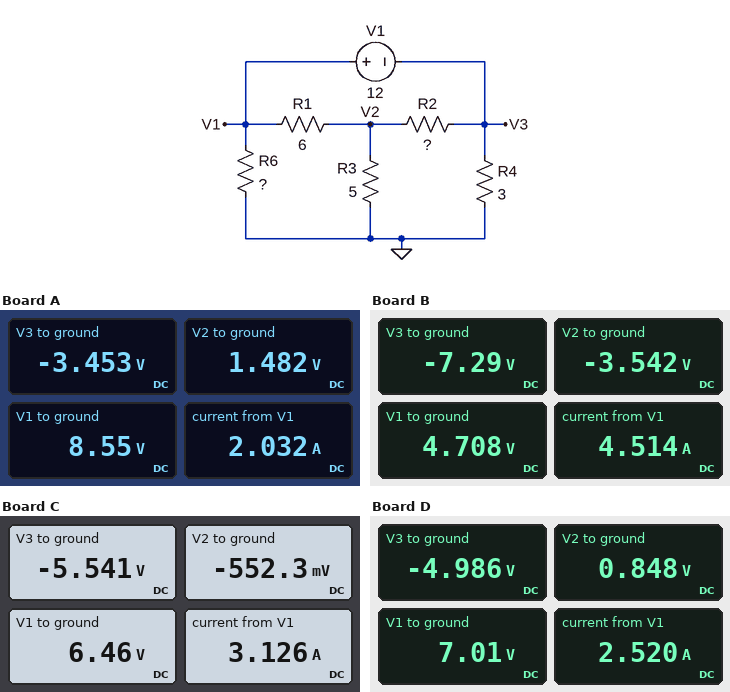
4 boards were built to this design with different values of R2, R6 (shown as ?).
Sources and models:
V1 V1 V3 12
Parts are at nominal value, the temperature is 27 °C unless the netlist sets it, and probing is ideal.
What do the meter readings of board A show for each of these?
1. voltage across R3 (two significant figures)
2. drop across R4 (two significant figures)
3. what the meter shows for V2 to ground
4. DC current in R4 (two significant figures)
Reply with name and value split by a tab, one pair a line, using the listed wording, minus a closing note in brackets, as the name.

voltage across R3	1.5 V
drop across R4	3.5 V
what the meter shows for V2 to ground	1.482 V
DC current in R4	1.2 A
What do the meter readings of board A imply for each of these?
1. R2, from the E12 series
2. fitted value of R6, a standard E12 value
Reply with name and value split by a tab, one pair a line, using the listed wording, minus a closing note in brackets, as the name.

R2, from the E12 series	5.6 Ω
fitted value of R6, a standard E12 value	10 Ω
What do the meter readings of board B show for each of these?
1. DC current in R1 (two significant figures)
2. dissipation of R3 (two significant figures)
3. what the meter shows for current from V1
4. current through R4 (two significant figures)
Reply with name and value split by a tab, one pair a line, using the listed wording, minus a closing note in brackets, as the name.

DC current in R1	1.4 A
dissipation of R3	2.5 W
what the meter shows for current from V1	4.514 A
current through R4	2.4 A
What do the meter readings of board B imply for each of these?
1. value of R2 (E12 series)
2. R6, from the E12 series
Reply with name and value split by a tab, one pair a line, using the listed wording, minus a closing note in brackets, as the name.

value of R2	1.8 Ω
R6, from the E12 series	1.5 Ω
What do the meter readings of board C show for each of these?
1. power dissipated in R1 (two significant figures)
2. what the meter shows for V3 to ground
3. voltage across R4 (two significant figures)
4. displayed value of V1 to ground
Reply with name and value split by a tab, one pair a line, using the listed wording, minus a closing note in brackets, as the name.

power dissipated in R1	8.2 W
what the meter shows for V3 to ground	-5.541 V
voltage across R4	5.5 V
displayed value of V1 to ground	6.46 V
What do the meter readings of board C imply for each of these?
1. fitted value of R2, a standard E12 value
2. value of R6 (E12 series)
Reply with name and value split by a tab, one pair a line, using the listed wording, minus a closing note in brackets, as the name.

fitted value of R2, a standard E12 value	3.9 Ω
value of R6	3.3 Ω
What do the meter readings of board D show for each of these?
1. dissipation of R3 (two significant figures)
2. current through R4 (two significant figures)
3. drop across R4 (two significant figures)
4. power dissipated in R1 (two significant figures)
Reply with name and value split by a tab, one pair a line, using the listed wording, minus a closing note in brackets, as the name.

dissipation of R3	140 mW
current through R4	1.7 A
drop across R4	5.0 V
power dissipated in R1	6.3 W
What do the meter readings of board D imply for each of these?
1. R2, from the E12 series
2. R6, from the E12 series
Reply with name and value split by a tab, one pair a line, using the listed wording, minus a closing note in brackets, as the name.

R2, from the E12 series	6.8 Ω
R6, from the E12 series	4.7 Ω
